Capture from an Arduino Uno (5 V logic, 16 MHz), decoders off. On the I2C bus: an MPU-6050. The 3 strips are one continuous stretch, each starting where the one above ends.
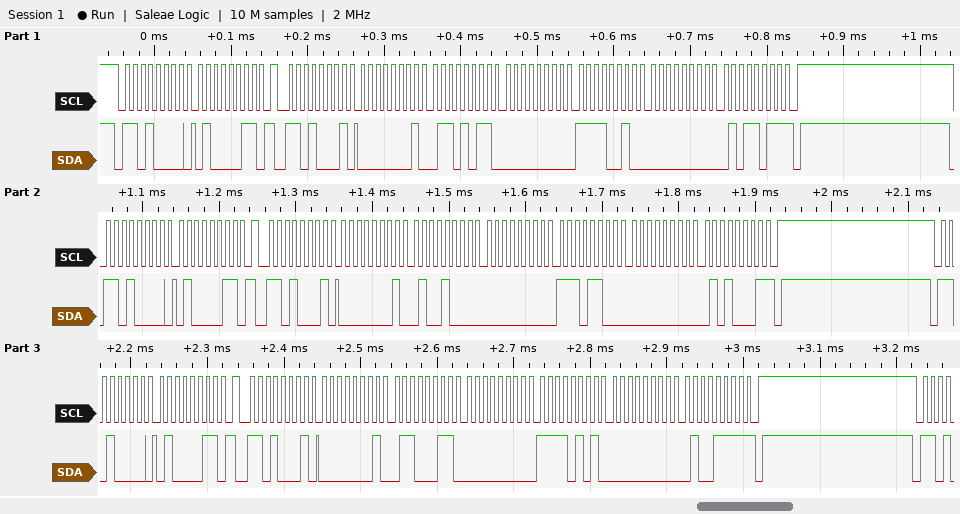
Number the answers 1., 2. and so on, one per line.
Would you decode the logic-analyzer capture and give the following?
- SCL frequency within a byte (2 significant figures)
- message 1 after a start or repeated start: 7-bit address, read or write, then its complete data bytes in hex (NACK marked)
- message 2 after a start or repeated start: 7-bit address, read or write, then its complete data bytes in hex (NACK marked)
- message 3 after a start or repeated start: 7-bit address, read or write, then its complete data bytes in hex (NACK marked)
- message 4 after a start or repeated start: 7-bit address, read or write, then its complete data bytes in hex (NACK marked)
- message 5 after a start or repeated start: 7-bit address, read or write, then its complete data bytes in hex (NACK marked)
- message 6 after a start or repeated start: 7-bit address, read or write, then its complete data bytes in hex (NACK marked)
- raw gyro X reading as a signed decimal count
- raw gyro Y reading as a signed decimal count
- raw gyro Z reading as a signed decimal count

1. 100 kHz
2. 0x68 write: 43
3. 0x68 read: 01 6B 00 F2 00 5B NACK
4. 0x68 write: 43
5. 0x68 read: 01 48 00 EC 00 51 NACK
6. 0x68 write: 43
7. 0x68 read: 01 63 00 F5 00 4F NACK
8. 363
9. 242
10. 91
